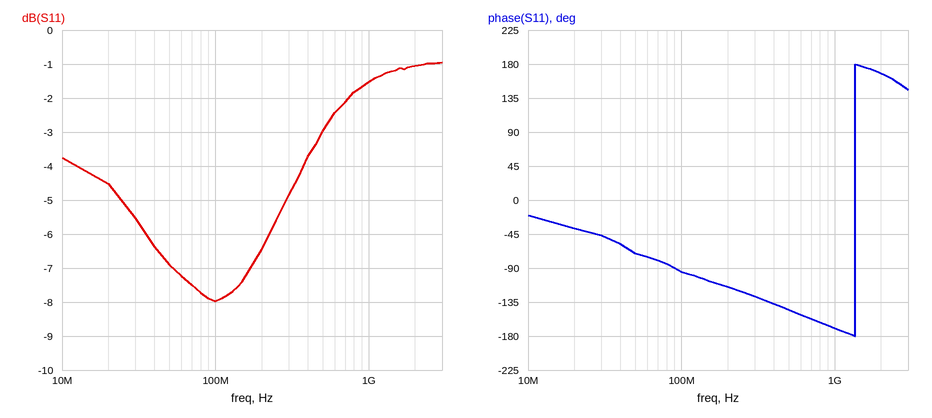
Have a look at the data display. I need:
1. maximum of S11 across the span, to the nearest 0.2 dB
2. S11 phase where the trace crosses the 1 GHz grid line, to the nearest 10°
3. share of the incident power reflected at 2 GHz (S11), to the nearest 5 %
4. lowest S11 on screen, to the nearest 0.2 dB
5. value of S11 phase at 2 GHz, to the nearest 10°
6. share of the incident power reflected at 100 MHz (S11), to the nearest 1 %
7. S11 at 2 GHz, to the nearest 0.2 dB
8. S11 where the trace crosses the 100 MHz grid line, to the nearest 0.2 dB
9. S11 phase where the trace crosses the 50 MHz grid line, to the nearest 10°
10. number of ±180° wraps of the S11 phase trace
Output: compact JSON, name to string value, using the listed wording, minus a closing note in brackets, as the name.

{"maximum of S11 across the span, to the nearest 0.2 dB": "-1.0 dB", "S11 phase where the trace crosses the 1 GHz grid line, to the nearest 10°": "-170°", "share of the incident power reflected at 2 GHz (S11), to the nearest 5 %": "80 %", "lowest S11 on screen, to the nearest 0.2 dB": "-8.0 dB", "value of S11 phase at 2 GHz, to the nearest 10°": "170°", "share of the incident power reflected at 100 MHz (S11), to the nearest 1 %": "16 %", "S11 at 2 GHz, to the nearest 0.2 dB": "-1.0 dB", "S11 where the trace crosses the 100 MHz grid line, to the nearest 0.2 dB": "-8.0 dB", "S11 phase where the trace crosses the 50 MHz grid line, to the nearest 10°": "-70°", "number of ±180° wraps of the S11 phase trace": "1"}
